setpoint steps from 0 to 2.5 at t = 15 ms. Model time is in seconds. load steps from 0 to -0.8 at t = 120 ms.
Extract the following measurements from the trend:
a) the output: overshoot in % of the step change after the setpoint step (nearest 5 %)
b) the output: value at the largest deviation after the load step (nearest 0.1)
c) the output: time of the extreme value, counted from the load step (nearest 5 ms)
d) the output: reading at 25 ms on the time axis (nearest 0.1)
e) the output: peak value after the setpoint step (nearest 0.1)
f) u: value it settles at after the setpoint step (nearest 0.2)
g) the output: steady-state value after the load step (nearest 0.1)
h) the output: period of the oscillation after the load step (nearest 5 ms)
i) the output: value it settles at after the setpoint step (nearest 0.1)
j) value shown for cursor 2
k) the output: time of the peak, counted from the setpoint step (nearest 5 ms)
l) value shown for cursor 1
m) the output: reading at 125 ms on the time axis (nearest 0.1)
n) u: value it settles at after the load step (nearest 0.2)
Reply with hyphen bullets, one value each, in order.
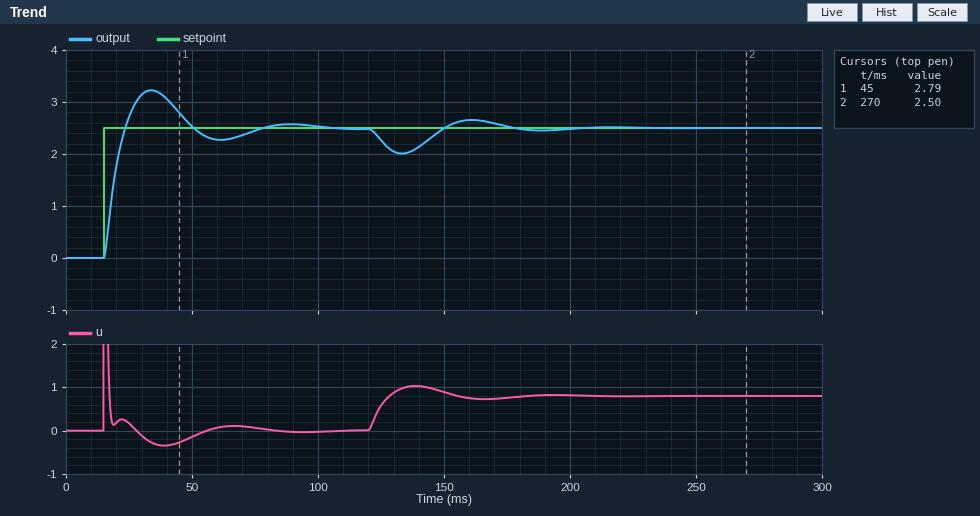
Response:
- 30 %
- 2.0
- 15 ms
- 2.7
- 3.2
- 0.0
- 2.5
- 55 ms
- 2.5
- 2.50
- 20 ms
- 2.79
- 2.3
- 0.8
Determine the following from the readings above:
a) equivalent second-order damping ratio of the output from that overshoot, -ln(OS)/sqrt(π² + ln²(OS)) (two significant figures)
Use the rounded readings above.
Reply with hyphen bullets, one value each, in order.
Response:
- 0.36
